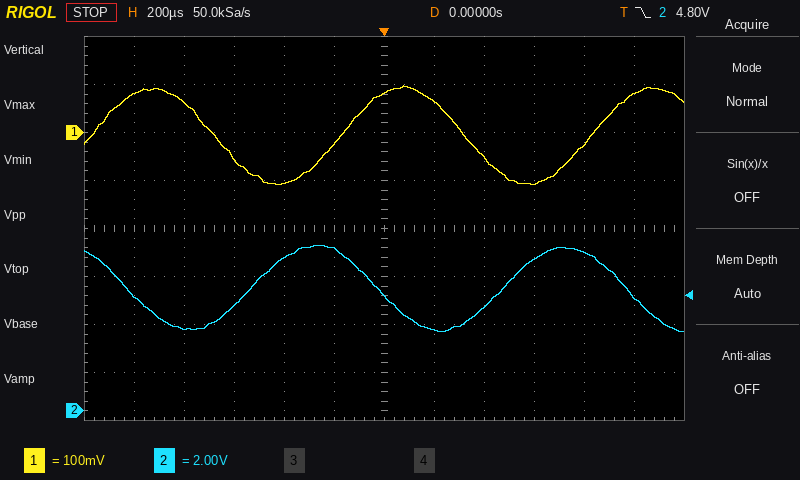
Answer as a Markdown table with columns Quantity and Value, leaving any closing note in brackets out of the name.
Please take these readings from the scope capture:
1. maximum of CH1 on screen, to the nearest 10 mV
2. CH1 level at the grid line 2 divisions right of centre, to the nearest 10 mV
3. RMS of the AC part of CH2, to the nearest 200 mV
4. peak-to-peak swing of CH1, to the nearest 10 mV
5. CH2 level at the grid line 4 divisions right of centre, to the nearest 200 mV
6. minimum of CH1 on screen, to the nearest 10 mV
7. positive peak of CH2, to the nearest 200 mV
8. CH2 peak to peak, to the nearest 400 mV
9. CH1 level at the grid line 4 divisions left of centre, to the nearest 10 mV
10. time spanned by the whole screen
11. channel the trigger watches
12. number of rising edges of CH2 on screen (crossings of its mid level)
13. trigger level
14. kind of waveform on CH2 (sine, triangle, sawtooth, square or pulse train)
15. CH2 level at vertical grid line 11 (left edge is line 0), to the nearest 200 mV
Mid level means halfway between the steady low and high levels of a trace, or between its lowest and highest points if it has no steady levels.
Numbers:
| Quantity | Value |
|---|---|
| maximum of CH1 on screen, to the nearest 10 mV | 100 mV |
| CH1 level at the grid line 2 divisions right of centre, to the nearest 10 mV | -50 mV |
| RMS of the AC part of CH2, to the nearest 200 mV | 1.2 V |
| peak-to-peak swing of CH1, to the nearest 10 mV | 210 mV |
| CH2 level at the grid line 4 divisions right of centre, to the nearest 200 mV | 6.6 V |
| minimum of CH1 on screen, to the nearest 10 mV | -110 mV |
| positive peak of CH2, to the nearest 200 mV | 6.8 V |
| CH2 peak to peak, to the nearest 400 mV | 3.6 V |
| CH1 level at the grid line 4 divisions left of centre, to the nearest 10 mV | 60 mV |
| time spanned by the whole screen | 2.4 ms |
| channel the trigger watches | CH2 |
| number of rising edges of CH2 on screen | 2 |
| trigger level | 4.80 V |
| kind of waveform on CH2 | sine |
| CH2 level at vertical grid line 11 (left edge is line 0), to the nearest 200 mV | 4.8 V |
